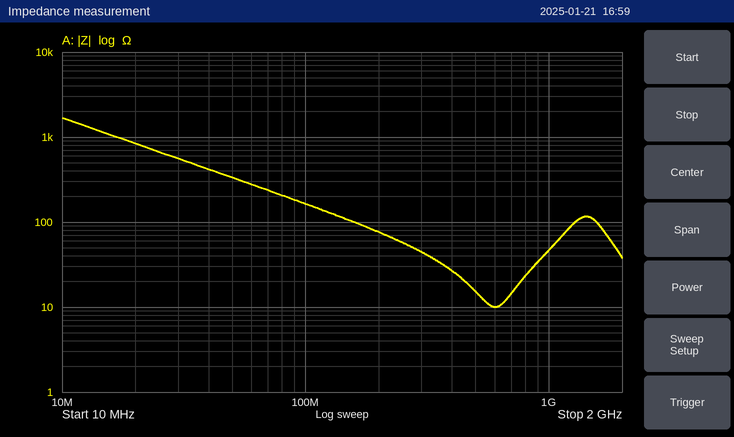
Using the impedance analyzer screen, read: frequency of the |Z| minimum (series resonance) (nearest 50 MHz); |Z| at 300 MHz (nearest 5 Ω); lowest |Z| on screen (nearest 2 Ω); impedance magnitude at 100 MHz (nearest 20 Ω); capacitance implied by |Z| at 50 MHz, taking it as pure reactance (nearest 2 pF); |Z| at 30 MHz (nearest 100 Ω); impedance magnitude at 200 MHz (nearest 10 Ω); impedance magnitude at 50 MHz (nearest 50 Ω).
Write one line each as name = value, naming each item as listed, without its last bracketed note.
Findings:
frequency of the |Z| minimum (series resonance) = 600 MHz
|Z| at 300 MHz = 45 Ω
lowest |Z| on screen = 10 Ω
impedance magnitude at 100 MHz = 160 Ω
capacitance implied by |Z| at 50 MHz, taking it as pure reactance = 10 pF
|Z| at 30 MHz = 600 Ω
impedance magnitude at 200 MHz = 80 Ω
impedance magnitude at 50 MHz = 350 Ω
